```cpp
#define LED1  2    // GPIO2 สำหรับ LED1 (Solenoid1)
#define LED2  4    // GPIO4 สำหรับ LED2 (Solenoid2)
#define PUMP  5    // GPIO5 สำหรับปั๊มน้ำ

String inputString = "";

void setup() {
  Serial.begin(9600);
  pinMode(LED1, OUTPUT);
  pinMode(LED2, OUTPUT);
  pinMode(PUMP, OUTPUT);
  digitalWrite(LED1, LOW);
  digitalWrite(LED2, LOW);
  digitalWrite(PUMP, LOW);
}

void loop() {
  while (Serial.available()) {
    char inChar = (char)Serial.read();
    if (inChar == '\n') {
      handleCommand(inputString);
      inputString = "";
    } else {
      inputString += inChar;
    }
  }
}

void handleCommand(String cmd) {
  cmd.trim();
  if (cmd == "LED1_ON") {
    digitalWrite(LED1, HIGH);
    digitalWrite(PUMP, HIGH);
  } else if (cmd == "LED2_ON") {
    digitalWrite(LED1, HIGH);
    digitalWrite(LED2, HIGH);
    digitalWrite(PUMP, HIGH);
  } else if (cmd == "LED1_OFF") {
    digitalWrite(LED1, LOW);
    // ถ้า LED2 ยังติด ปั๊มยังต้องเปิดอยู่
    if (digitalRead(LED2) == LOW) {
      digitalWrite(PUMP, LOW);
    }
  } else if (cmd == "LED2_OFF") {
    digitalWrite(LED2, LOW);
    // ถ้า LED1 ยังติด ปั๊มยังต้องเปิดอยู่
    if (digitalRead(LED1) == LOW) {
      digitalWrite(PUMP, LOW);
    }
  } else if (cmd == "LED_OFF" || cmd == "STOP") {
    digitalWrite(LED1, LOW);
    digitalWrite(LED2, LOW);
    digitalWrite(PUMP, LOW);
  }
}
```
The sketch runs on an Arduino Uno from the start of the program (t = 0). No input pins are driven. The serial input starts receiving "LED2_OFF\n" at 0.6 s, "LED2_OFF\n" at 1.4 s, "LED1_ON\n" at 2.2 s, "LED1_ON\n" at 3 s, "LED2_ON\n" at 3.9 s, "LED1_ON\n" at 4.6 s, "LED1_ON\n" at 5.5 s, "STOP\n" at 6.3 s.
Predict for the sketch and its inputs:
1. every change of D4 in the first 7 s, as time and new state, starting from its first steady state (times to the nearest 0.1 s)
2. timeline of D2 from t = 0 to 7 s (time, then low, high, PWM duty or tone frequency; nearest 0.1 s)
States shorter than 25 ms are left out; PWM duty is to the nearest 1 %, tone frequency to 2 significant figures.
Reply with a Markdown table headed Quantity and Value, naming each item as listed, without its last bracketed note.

| Quantity | Value |
|---|---|
| every change of D4 in the first 7 s, as time and new state, starting from its first steady state | 0 s low; 3.9 s high; 6.3 s low |
| timeline of D2 from t = 0 to 7 s | 0 s low; 2.2 s high; 6.3 s low |
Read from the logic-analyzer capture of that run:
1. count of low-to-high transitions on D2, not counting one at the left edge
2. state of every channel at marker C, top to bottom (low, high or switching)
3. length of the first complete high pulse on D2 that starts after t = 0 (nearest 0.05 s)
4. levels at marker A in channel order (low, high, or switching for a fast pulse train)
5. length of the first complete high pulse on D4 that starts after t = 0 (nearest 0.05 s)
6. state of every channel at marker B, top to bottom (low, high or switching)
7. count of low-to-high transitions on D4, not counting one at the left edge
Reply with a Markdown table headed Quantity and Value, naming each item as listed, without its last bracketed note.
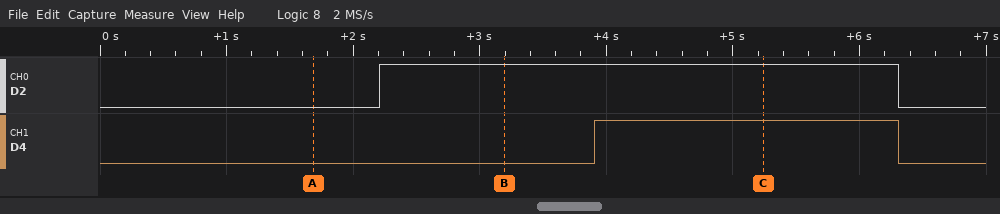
| Quantity | Value |
|---|---|
| count of low-to-high transitions on D2, not counting one at the left edge | 1 |
| state of every channel at marker C, top to bottom | D2 high, D4 high |
| length of the first complete high pulse on D2 that starts after t = 0 | 4.10 s |
| levels at marker A in channel order | D2 low, D4 low |
| length of the first complete high pulse on D4 that starts after t = 0 | 2.40 s |
| state of every channel at marker B, top to bottom | D2 high, D4 low |
| count of low-to-high transitions on D4, not counting one at the left edge | 1 |
